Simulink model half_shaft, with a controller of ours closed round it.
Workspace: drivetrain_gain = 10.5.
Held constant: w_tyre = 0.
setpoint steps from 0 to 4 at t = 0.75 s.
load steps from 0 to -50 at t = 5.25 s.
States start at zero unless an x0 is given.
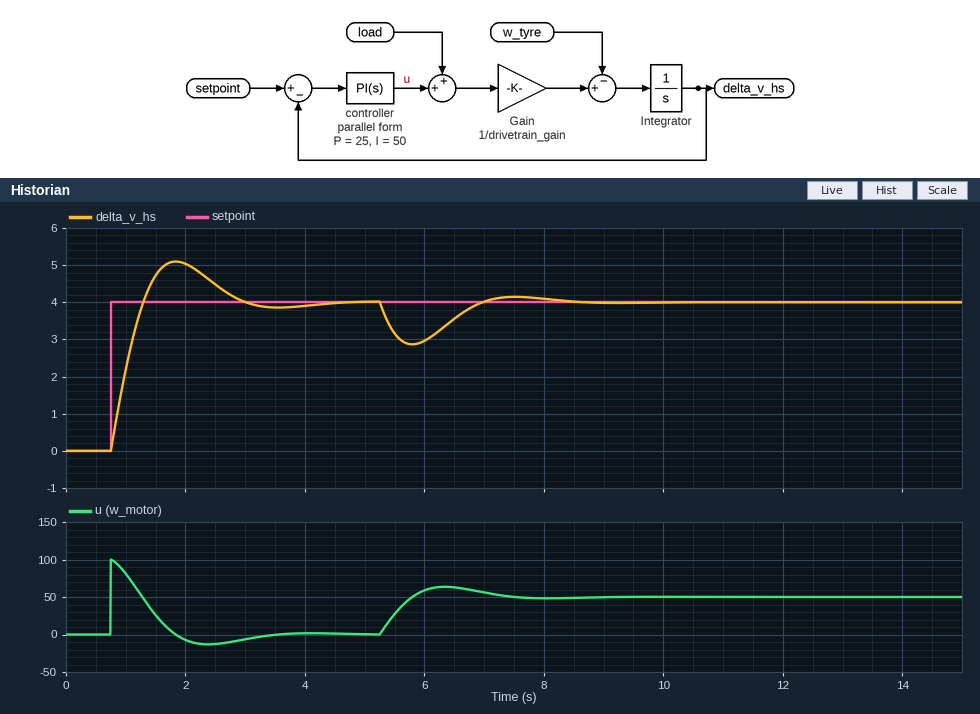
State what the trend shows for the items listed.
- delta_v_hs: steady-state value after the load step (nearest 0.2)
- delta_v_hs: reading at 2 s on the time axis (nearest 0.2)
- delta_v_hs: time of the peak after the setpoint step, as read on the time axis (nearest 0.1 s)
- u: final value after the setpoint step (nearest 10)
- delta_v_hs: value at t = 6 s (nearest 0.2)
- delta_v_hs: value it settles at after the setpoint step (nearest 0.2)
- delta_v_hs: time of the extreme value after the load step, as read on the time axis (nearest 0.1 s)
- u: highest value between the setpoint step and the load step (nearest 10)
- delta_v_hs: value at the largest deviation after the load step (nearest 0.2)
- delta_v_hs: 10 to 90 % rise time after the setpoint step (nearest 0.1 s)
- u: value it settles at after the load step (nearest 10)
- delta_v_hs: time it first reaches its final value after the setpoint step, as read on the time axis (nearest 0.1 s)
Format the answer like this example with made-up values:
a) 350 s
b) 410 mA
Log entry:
a) 4.0
b) 5.0
c) 1.8 s
d) 0
e) 3.0
f) 4.0
g) 5.8 s
h) 100
i) 2.8
j) 0.4 s
k) 50
l) 1.3 s
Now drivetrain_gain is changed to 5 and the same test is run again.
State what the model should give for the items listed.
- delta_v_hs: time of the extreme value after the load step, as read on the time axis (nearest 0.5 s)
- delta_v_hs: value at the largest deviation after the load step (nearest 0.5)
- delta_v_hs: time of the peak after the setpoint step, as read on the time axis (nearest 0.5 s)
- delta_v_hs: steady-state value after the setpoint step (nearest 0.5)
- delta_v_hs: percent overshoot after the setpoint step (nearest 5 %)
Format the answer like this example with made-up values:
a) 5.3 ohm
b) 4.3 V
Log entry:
a) 5.5 s
b) 2.5
c) 1.5 s
d) 4.0
e) 20 %
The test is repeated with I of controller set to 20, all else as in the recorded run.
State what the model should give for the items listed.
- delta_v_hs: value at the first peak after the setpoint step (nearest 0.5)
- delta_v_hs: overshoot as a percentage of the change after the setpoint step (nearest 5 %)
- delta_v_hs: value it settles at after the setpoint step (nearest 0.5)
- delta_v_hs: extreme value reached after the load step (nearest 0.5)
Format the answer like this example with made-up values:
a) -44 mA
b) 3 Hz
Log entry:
a) 4.5
b) 15 %
c) 4.0
d) 2.5
